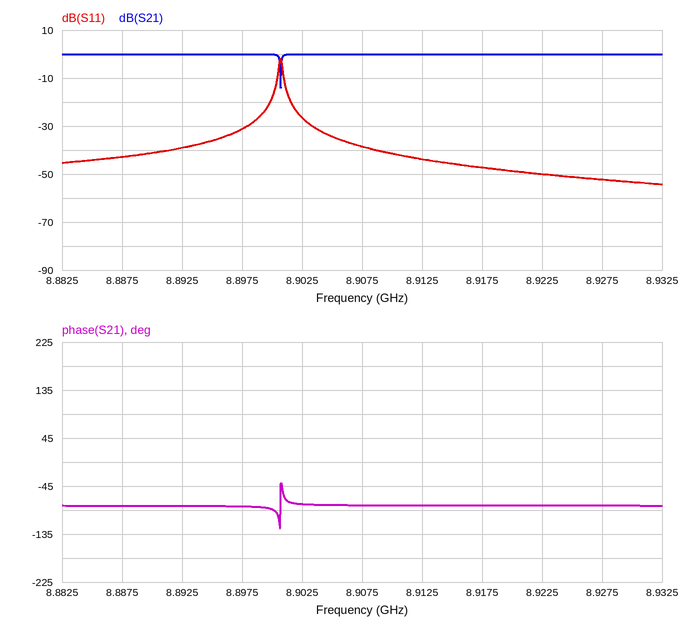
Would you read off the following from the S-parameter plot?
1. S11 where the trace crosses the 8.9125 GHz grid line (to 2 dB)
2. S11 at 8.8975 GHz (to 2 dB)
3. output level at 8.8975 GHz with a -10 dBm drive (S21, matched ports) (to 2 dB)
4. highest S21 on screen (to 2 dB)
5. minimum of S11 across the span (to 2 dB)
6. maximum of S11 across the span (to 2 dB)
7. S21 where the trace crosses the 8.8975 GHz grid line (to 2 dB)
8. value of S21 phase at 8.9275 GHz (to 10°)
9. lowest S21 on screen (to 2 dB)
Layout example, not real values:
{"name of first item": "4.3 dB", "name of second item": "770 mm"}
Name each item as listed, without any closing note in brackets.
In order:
{"S11 where the trace crosses the 8.9125 GHz grid line": "-44 dB", "S11 at 8.8975 GHz": "-32 dB", "output level at 8.8975 GHz with a -10 dBm drive (S21, matched ports)": "-10 dBm", "highest S21 on screen": "0 dB", "minimum of S11 across the span": "-54 dB", "maximum of S11 across the span": "-2 dB", "S21 where the trace crosses the 8.8975 GHz grid line": "0 dB", "value of S21 phase at 8.9275 GHz": "-80°", "lowest S21 on screen": "-14 dB"}
